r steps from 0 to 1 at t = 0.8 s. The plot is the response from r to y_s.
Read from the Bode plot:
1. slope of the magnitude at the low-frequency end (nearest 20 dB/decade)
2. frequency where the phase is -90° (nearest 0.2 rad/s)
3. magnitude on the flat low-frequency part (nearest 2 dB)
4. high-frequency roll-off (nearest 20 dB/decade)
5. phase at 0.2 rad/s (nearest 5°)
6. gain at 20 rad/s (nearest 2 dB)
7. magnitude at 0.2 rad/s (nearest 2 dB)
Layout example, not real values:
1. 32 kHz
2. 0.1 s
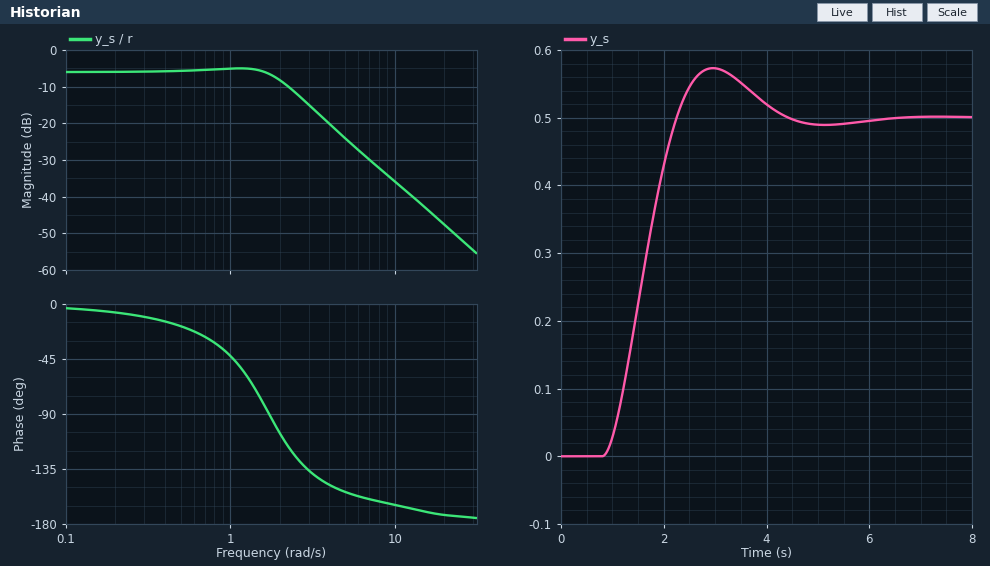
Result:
1. 0 dB/decade
2. 1.8 rad/s
3. -6 dB
4. -40 dB/decade
5. -5°
6. -48 dB
7. -6 dB
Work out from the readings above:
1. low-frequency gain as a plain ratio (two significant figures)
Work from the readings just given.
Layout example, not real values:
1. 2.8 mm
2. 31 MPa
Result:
1. 0.50
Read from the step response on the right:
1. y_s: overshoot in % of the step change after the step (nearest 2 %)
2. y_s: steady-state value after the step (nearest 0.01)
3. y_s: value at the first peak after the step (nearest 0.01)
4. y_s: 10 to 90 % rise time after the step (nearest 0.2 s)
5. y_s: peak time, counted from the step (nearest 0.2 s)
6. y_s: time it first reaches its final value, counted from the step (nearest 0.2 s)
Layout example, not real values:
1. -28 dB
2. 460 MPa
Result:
1. 14 %
2. 0.50
3. 0.57
4. 1.0 s
5. 2.2 s
6. 1.4 s
